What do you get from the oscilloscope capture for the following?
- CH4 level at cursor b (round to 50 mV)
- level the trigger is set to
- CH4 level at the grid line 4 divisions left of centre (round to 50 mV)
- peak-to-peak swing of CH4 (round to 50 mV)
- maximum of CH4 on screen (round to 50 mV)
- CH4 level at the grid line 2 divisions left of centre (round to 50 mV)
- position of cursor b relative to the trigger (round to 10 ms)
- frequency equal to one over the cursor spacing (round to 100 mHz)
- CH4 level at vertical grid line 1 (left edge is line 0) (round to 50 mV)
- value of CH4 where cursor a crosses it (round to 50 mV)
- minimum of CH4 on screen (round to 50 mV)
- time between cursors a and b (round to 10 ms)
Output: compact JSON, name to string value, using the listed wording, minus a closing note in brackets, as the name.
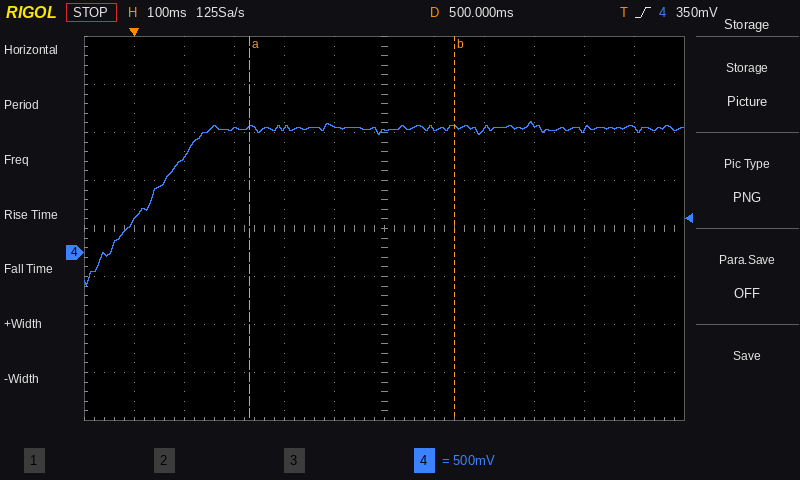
{"CH4 level at cursor b": "1.30 V", "level the trigger is set to": "350 mV", "CH4 level at the grid line 4 divisions left of centre": "1.00 V", "peak-to-peak swing of CH4": "1.70 V", "maximum of CH4 on screen": "1.35 V", "CH4 level at the grid line 2 divisions left of centre": "1.30 V", "position of cursor b relative to the trigger": "+640 ms", "frequency equal to one over the cursor spacing": "2.4 Hz", "CH4 level at vertical grid line 1 (left edge is line 0)": "350 mV", "value of CH4 where cursor a crosses it": "1.30 V", "minimum of CH4 on screen": "-350 mV", "time between cursors a and b": "410 ms"}
